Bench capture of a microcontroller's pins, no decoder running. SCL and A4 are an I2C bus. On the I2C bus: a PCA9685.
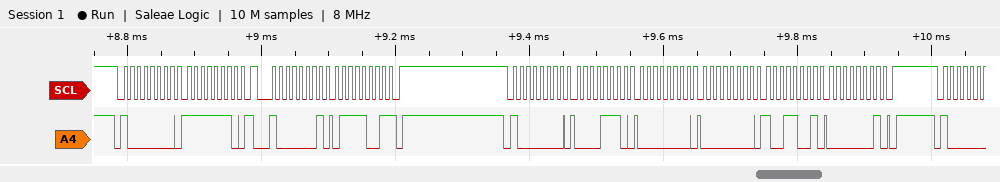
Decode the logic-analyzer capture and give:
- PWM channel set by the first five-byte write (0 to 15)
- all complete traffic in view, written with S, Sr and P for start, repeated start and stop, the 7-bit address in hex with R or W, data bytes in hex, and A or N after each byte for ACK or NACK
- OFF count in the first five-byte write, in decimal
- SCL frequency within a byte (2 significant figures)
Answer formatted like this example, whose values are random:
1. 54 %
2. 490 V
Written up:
1. 2
2. S 40W A FE A Sr 40R A 79 N P S 40W A 0E A 00 A 00 A 99 A 01 A P
3. 409
4. 100 kHz
